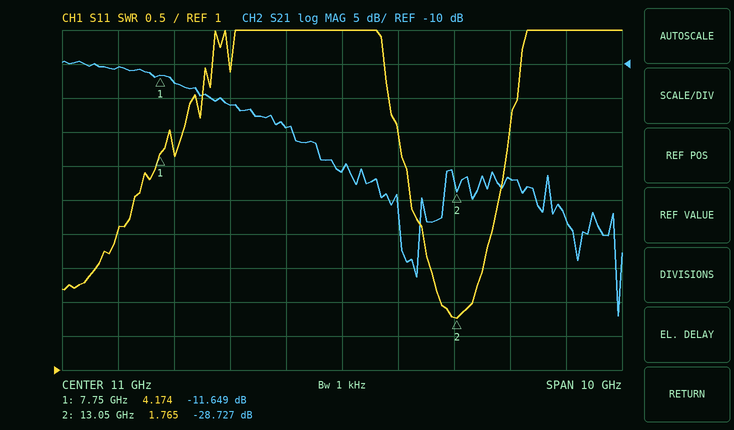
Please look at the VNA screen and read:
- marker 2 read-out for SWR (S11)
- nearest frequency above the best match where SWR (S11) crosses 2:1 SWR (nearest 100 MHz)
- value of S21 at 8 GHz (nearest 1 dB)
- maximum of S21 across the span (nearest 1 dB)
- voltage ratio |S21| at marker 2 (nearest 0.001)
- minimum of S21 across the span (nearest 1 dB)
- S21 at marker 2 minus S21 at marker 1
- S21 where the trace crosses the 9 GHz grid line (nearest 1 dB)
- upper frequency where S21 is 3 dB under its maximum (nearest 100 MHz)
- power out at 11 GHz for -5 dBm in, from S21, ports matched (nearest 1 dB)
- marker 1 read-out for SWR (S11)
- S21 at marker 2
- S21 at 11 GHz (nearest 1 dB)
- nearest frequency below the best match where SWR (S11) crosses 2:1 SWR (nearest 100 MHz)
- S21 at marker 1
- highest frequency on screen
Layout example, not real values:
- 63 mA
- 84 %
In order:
- 1.765
- 13.3 GHz
- -13 dB
- -10 dB
- 0.037
- -47 dB
- -17.078 dB
- -16 dB
- 8.0 GHz
- -31 dBm
- 4.174
- -28.727 dB
- -26 dB
- 12.8 GHz
- -11.649 dB
- 16 GHz
